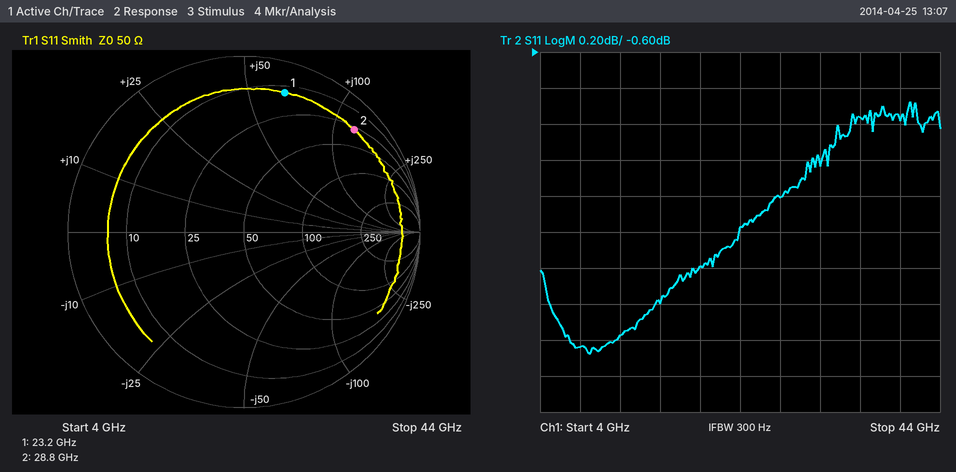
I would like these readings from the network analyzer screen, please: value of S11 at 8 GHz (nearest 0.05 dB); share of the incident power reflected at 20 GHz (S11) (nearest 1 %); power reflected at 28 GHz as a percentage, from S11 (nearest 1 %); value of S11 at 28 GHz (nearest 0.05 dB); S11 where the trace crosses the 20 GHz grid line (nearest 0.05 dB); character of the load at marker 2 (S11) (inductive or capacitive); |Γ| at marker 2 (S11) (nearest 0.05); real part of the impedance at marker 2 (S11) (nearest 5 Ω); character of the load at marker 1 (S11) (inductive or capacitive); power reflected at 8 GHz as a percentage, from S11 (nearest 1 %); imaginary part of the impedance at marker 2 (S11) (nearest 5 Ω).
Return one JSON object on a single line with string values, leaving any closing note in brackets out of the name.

{"value of S11 at 8 GHz": "-2.25 dB", "share of the incident power reflected at 20 GHz (S11)": "66 %", "power reflected at 28 GHz as a percentage, from S11": "72 %", "value of S11 at 28 GHz": "-1.40 dB", "S11 where the trace crosses the 20 GHz grid line": "-1.80 dB", "character of the load at marker 2 (S11)": "inductive", "|Γ| at marker 2 (S11)": "0.85", "real part of the impedance at marker 2 (S11)": "30 Ω", "character of the load at marker 1 (S11)": "inductive", "power reflected at 8 GHz as a percentage, from S11": "60 %", "imaginary part of the impedance at marker 2 (S11)": "+120 Ω"}
